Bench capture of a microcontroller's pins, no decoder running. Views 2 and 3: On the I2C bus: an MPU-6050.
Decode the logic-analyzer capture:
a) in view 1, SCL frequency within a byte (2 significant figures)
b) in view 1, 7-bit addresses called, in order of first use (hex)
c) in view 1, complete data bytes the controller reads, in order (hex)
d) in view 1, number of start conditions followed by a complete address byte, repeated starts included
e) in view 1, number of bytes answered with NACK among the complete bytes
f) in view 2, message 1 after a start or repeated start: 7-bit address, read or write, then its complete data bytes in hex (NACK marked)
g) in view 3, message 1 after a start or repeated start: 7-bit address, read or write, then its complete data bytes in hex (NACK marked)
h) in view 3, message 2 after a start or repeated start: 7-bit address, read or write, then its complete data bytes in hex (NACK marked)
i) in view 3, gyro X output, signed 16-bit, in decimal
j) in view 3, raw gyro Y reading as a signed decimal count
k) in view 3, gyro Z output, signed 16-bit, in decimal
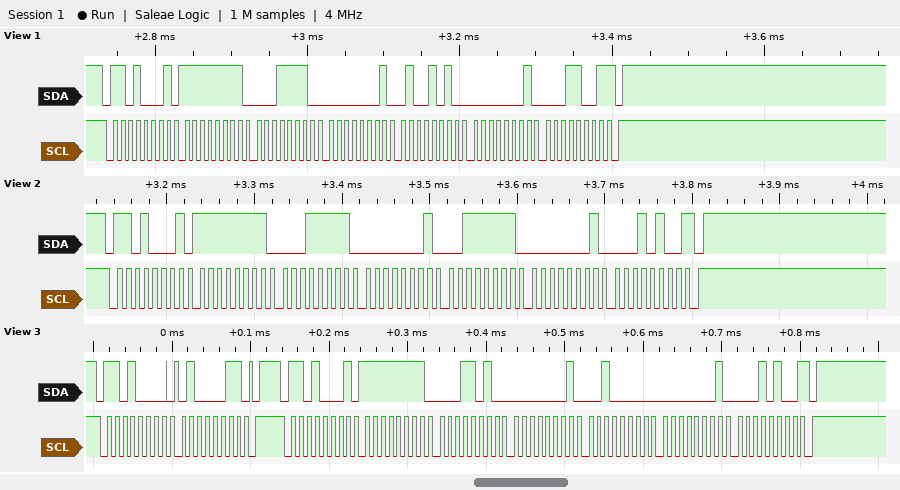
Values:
100 kHz
0x68
FF 1E 01 4A 01 19
1
1
0x68 read: FF 1F 01 3F 01 14 NACK
0x68 write: 43
0x68 read: FF 1A 01 20 01 14 NACK
-230
288
276
